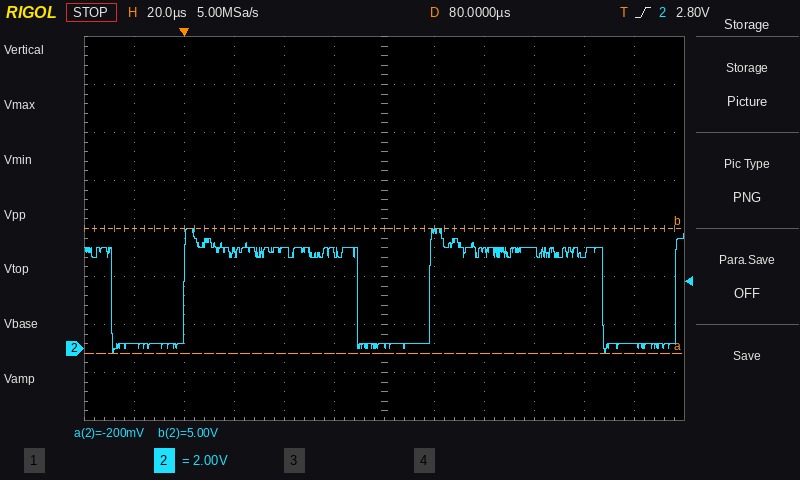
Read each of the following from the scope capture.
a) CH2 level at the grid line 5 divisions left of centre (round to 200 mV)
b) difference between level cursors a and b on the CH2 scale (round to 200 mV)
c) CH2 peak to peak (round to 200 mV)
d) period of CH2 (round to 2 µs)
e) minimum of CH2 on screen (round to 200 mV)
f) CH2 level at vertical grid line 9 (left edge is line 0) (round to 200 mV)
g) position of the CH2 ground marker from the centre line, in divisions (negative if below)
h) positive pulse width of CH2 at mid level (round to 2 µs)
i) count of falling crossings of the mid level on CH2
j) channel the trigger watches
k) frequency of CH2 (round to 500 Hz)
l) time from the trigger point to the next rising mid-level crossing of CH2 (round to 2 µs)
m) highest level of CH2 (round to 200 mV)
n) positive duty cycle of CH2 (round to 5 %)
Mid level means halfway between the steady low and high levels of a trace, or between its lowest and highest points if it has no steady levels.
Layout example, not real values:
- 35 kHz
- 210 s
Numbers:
- 200 mV
- 5.2 V
- 5.2 V
- 98 µs
- -200 mV
- 4.0 V
- -2.5 div
- 70 µs
- 3
- CH2
- 10.0 kHz
- 98 µs
- 5.0 V
- 70 %
